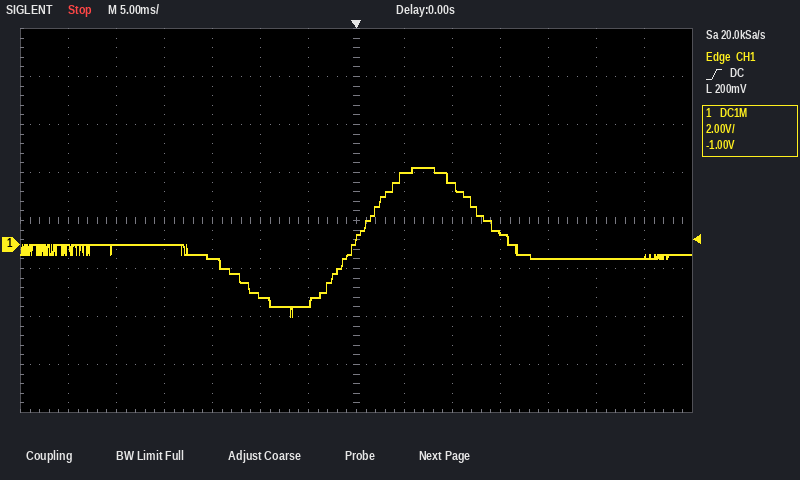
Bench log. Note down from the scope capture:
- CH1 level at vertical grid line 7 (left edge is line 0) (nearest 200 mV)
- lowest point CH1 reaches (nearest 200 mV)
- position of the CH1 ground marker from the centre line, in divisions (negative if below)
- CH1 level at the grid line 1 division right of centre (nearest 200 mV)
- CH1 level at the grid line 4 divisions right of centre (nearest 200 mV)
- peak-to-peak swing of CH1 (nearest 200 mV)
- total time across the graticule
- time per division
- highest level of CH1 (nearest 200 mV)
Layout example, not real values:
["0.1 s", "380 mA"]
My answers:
["200 mV", "-3.0 V", "-0.5 div", "3.0 V", "-600 mV", "6.2 V", "70 ms", "5 ms", "3.2 V"]
